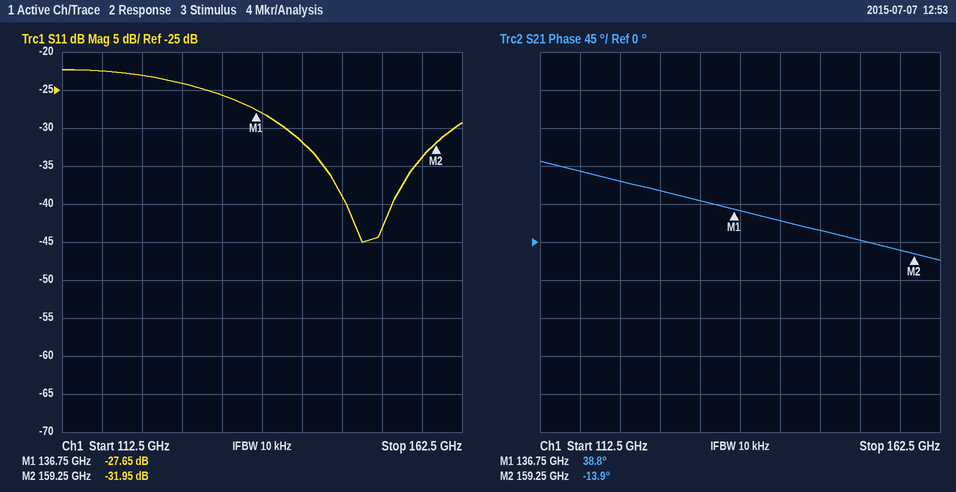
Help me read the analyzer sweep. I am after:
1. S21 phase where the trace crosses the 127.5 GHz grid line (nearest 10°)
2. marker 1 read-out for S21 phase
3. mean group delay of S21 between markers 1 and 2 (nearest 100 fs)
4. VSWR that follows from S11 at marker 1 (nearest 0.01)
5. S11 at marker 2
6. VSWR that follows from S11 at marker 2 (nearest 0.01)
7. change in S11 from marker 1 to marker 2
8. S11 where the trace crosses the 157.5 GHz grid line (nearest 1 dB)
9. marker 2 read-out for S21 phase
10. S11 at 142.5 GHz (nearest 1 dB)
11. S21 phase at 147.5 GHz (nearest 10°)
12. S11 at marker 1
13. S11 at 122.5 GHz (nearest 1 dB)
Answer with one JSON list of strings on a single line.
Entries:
["60°", "38.8°", "6.5 ps", "1.09", "-31.95 dB", "1.05", "-4.30 dB", "-34 dB", "-13.9°", "-32 dB", "10°", "-27.65 dB", "-23 dB"]
